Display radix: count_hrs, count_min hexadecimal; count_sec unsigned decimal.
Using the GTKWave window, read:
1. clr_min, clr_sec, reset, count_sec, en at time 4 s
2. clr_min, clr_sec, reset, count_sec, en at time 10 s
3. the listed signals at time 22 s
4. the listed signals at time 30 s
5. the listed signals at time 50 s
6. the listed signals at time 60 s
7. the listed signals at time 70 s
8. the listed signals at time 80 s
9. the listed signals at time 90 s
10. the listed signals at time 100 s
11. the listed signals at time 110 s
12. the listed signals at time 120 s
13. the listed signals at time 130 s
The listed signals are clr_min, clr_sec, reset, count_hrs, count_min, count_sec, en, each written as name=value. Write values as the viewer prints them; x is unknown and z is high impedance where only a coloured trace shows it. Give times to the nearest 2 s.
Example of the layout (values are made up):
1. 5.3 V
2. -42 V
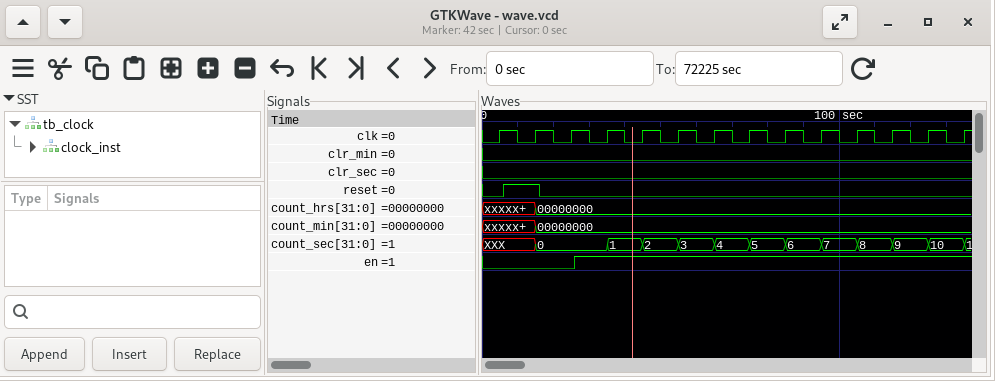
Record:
1. clr_min=0, clr_sec=0, reset=0, count_sec=XXX, en=0
2. clr_min=0, clr_sec=0, reset=1, count_sec=XXX, en=0
3. clr_min=0, clr_sec=0, reset=0, count_hrs=00000000, count_min=00000000, count_sec=0, en=0
4. clr_min=0, clr_sec=0, reset=0, count_hrs=00000000, count_min=00000000, count_sec=0, en=1
5. clr_min=0, clr_sec=0, reset=0, count_hrs=00000000, count_min=00000000, count_sec=2, en=1
6. clr_min=0, clr_sec=0, reset=0, count_hrs=00000000, count_min=00000000, count_sec=3, en=1
7. clr_min=0, clr_sec=0, reset=0, count_hrs=00000000, count_min=00000000, count_sec=4, en=1
8. clr_min=0, clr_sec=0, reset=0, count_hrs=00000000, count_min=00000000, count_sec=5, en=1
9. clr_min=0, clr_sec=0, reset=0, count_hrs=00000000, count_min=00000000, count_sec=6, en=1
10. clr_min=0, clr_sec=0, reset=0, count_hrs=00000000, count_min=00000000, count_sec=7, en=1
11. clr_min=0, clr_sec=0, reset=0, count_hrs=00000000, count_min=00000000, count_sec=8, en=1
12. clr_min=0, clr_sec=0, reset=0, count_hrs=00000000, count_min=00000000, count_sec=9, en=1
13. clr_min=0, clr_sec=0, reset=0, count_hrs=00000000, count_min=00000000, count_sec=10, en=1
